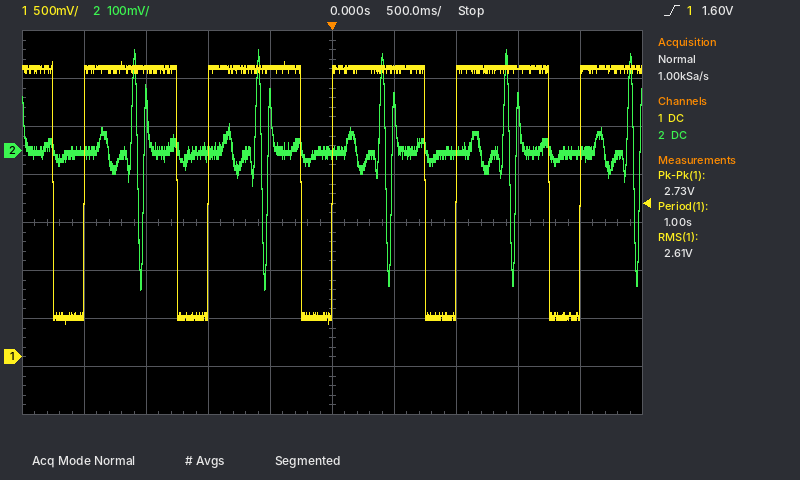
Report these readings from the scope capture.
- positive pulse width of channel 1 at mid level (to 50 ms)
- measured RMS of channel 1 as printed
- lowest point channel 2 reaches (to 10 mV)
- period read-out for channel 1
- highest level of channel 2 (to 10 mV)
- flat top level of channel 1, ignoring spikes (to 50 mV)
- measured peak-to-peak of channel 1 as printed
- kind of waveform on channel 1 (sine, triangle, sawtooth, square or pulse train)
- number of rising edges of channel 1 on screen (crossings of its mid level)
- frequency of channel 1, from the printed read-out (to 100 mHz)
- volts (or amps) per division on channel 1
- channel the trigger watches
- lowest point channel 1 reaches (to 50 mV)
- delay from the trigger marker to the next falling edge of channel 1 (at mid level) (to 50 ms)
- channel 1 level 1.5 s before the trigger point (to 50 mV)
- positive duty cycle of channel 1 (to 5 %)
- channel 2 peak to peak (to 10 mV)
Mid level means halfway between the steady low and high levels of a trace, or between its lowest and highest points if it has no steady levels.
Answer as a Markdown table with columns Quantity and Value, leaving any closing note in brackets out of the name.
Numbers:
| Quantity | Value |
|---|---|
| positive pulse width of channel 1 at mid level | 750 ms |
| measured RMS of channel 1 as printed | 2.61 V |
| lowest point channel 2 reaches | -290 mV |
| period read-out for channel 1 | 1.00 s |
| highest level of channel 2 | 210 mV |
| flat top level of channel 1, ignoring spikes | 3.00 V |
| measured peak-to-peak of channel 1 as printed | 2.73 V |
| kind of waveform on channel 1 | pulse train |
| number of rising edges of channel 1 on screen | 5 |
| frequency of channel 1, from the printed read-out | 1.0 Hz |
| volts (or amps) per division on channel 1 | 500 mV |
| channel the trigger watches | channel 1 |
| lowest point channel 1 reaches | 350 mV |
| delay from the trigger marker to the next falling edge of channel 1 (at mid level) | 750 ms |
| channel 1 level 1.5 s before the trigger point | 3.00 V |
| positive duty cycle of channel 1 | 75 % |
| channel 2 peak to peak | 500 mV |
